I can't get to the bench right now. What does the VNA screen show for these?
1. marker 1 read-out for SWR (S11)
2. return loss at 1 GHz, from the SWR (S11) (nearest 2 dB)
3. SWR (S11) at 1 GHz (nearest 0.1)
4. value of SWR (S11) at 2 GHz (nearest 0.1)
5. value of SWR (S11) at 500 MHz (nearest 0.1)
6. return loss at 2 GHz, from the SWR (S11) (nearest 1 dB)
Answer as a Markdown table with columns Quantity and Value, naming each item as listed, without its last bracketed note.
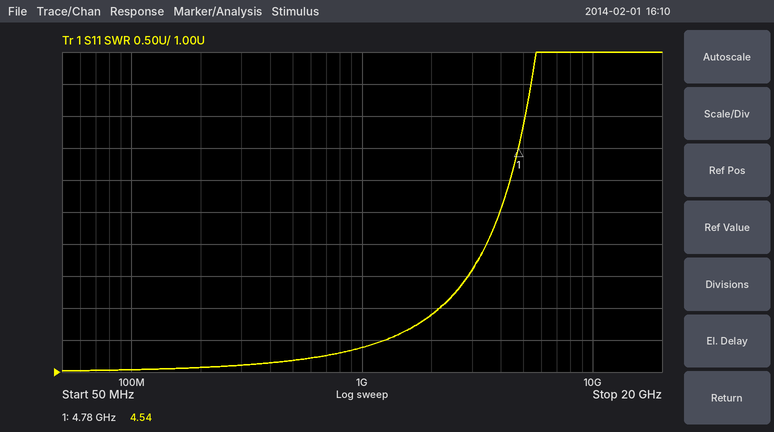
| Quantity | Value |
|---|---|
| marker 1 read-out for SWR | 4.54 |
| return loss at 1 GHz, from the SWR (S11) | 16 dB |
| SWR (S11) at 1 GHz | 1.4 |
| value of SWR (S11) at 2 GHz | 1.9 |
| value of SWR (S11) at 500 MHz | 1.2 |
| return loss at 2 GHz, from the SWR (S11) | 10 dB |
